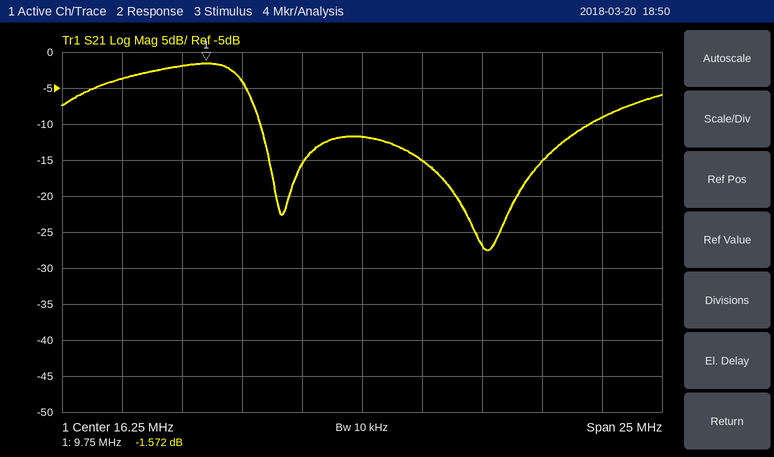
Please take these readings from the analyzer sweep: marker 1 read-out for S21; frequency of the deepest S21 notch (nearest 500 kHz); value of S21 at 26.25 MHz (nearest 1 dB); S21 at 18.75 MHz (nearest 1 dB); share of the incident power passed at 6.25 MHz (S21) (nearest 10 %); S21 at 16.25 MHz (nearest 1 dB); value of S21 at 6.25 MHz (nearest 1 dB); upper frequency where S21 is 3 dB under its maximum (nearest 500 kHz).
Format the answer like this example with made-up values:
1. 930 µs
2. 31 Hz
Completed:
1. -1.572 dB
2. 21.5 MHz
3. -9 dB
4. -15 dB
5. 40 %
6. -12 dB
7. -4 dB
8. 11.5 MHz
